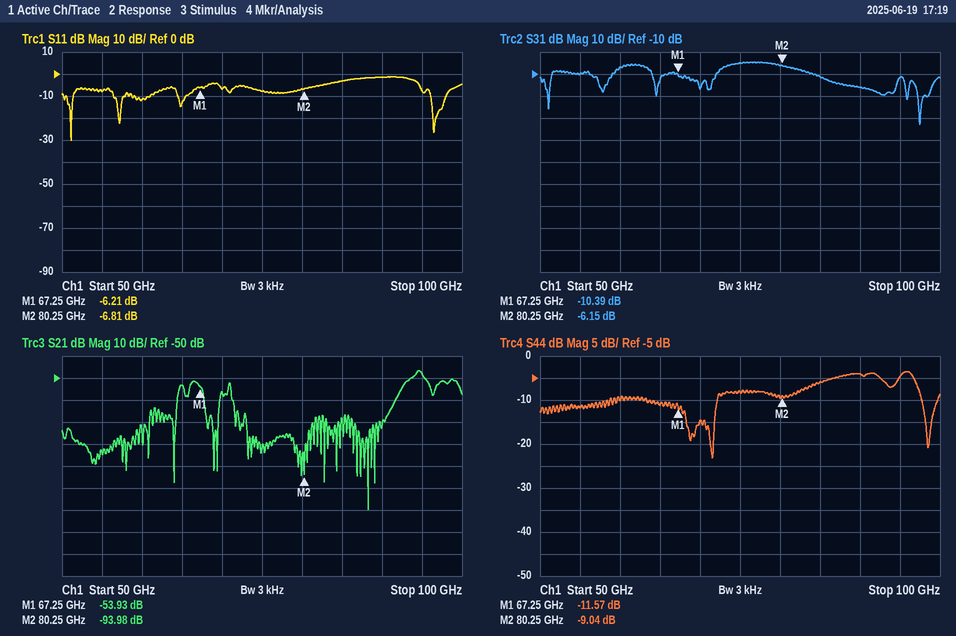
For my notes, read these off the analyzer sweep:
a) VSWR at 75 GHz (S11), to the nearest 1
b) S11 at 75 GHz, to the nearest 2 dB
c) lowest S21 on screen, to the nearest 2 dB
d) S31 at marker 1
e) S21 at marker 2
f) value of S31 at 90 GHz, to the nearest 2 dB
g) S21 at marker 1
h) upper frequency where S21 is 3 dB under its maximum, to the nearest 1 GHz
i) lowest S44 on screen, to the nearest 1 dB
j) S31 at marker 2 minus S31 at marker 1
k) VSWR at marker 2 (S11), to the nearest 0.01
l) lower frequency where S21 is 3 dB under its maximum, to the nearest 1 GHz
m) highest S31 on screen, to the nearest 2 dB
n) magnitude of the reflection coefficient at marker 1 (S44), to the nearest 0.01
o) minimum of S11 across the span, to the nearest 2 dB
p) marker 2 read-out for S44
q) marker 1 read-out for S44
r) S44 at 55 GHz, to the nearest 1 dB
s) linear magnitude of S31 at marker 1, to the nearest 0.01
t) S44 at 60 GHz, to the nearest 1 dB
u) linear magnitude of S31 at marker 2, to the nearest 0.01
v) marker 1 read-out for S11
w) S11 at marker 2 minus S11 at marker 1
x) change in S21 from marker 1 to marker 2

2
-8 dB
-110 dB
-10.39 dB
-93.98 dB
-16 dB
-53.93 dB
95 GHz
-23 dB
4.24 dB
2.68
94 GHz
-4 dB
0.26
-30 dB
-9.04 dB
-11.57 dB
-12 dB
0.30
-10 dB
0.49
-6.21 dB
-0.60 dB
-40.05 dB
